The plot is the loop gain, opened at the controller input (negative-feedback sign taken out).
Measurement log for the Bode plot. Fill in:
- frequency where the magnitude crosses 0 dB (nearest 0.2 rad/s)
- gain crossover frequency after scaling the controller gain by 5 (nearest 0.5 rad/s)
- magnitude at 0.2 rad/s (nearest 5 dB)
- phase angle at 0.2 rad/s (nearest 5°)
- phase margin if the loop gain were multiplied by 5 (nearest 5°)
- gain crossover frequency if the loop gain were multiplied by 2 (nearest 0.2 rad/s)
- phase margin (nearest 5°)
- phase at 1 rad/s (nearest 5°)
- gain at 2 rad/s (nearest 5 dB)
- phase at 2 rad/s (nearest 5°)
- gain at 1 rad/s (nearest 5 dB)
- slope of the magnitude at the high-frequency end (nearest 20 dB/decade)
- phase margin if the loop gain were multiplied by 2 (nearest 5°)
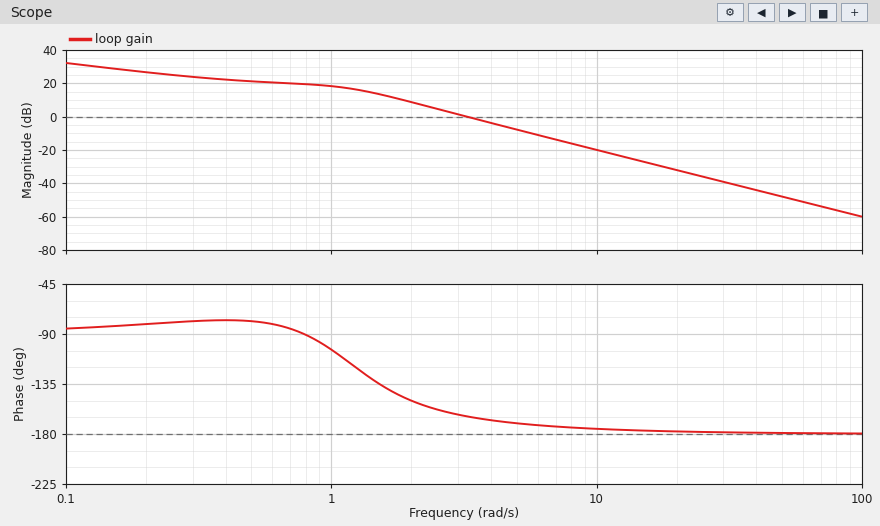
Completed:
3.2 rad/s
7.0 rad/s
25 dB
-80°
5°
4.6 rad/s
15°
-105°
10 dB
-150°
20 dB
-40 dB/decade
10°
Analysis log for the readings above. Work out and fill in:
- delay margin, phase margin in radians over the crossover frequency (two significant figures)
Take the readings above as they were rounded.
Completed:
0.082 s
